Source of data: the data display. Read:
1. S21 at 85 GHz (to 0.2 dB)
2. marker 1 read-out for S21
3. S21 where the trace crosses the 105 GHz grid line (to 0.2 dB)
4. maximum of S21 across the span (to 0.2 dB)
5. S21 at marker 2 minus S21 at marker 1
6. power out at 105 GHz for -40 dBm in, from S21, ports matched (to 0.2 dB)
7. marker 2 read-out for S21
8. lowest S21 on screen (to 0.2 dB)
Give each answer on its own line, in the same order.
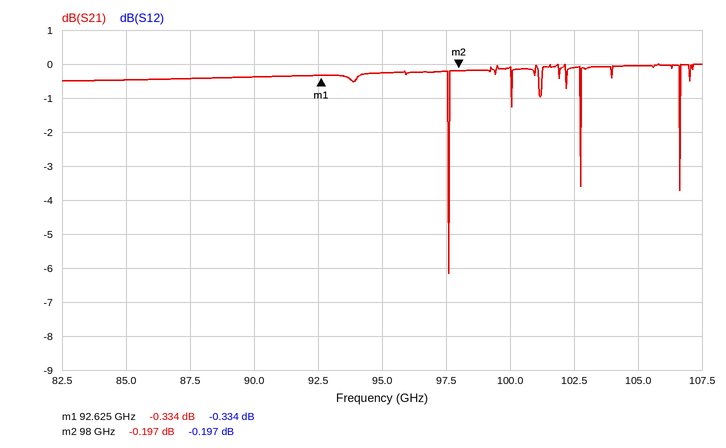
-0.4 dB
-0.334 dB
0.0 dB
0.0 dB
0.137 dB
-40.0 dBm
-0.197 dB
-6.2 dB
